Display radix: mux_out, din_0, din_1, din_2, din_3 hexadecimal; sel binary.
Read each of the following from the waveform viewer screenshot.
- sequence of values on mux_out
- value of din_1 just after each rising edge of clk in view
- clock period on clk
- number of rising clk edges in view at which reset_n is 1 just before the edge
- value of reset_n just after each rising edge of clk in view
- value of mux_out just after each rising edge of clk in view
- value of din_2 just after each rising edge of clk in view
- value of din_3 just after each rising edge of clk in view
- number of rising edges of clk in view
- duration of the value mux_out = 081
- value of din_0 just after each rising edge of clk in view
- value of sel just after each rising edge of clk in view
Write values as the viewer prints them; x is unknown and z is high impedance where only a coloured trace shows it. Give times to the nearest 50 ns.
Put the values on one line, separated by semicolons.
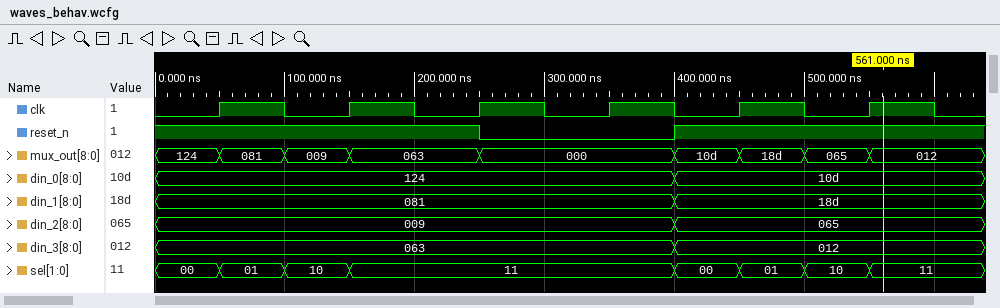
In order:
124, 081, 009, 063, 000, 10d, 18d, 065, 012; 081, 081, 081, 081, 18d, 18d; 100 ns; 5; 1 1 0 0 1 1; 081, 063, 000, 000, 18d, 012; 009, 009, 009, 009, 065, 065; 063, 063, 063, 063, 012, 012; 6; 50 ns; 124, 124, 124, 124, 10d, 10d; 01, 11, 11, 11, 01, 11
